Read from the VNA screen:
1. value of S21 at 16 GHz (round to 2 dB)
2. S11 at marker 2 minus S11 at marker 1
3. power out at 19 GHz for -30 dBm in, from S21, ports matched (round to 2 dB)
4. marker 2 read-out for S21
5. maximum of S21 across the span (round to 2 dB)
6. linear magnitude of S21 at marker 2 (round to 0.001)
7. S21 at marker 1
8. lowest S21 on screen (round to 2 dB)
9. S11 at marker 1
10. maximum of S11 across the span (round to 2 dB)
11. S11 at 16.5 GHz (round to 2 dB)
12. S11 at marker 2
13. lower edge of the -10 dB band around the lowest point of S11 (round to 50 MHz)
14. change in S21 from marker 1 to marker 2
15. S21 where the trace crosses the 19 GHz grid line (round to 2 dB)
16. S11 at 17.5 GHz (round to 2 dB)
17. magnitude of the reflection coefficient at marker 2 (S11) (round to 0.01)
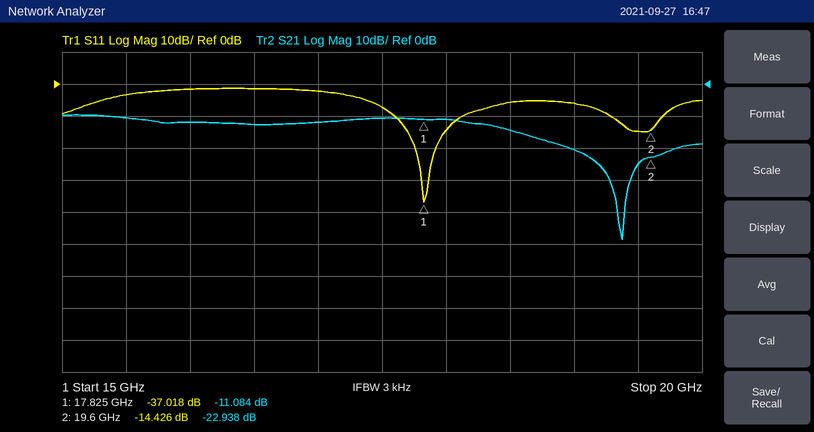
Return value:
-12 dB
22.592 dB
-50 dBm
-22.938 dB
-10 dB
0.071
-11.084 dB
-48 dB
-37.018 dB
-2 dB
-2 dB
-14.426 dB
17.60 GHz
-11.854 dB
-20 dB
-8 dB
0.19
